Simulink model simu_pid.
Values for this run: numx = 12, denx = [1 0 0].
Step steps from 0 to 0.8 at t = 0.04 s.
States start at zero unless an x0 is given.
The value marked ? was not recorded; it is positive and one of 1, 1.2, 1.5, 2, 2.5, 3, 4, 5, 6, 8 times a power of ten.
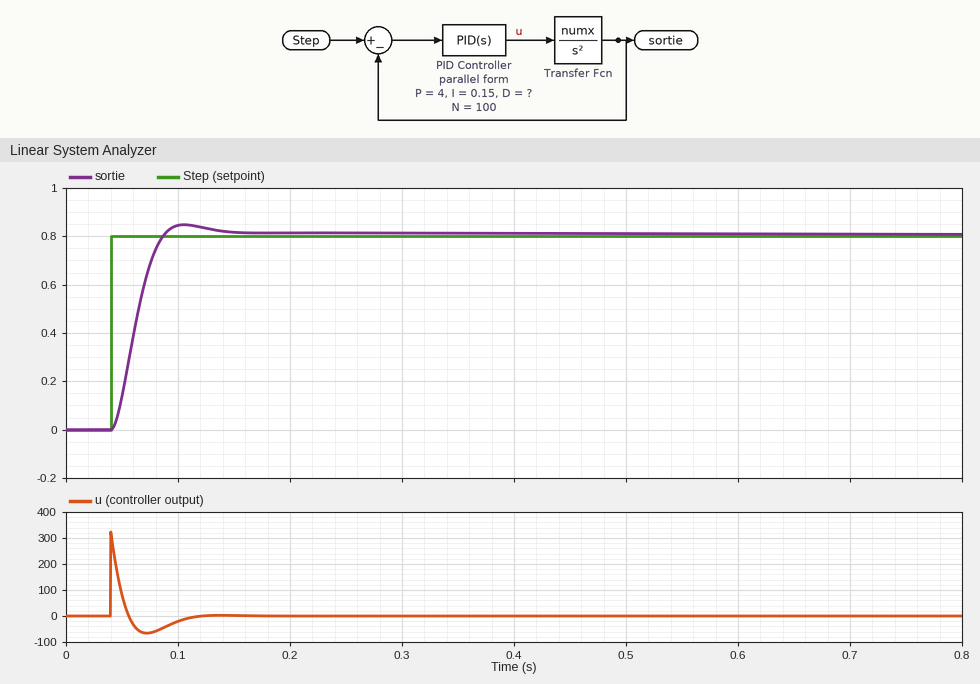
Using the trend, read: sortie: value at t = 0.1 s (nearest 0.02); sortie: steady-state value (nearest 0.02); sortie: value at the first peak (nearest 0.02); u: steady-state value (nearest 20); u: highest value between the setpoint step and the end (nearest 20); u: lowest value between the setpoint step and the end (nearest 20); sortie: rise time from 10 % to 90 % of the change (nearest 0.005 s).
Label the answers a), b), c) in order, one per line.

a) 0.84
b) 0.80
c) 0.84
d) 0
e) 320
f) -60
g) 0.030 s
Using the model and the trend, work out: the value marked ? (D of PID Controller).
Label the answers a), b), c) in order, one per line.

a) 4
